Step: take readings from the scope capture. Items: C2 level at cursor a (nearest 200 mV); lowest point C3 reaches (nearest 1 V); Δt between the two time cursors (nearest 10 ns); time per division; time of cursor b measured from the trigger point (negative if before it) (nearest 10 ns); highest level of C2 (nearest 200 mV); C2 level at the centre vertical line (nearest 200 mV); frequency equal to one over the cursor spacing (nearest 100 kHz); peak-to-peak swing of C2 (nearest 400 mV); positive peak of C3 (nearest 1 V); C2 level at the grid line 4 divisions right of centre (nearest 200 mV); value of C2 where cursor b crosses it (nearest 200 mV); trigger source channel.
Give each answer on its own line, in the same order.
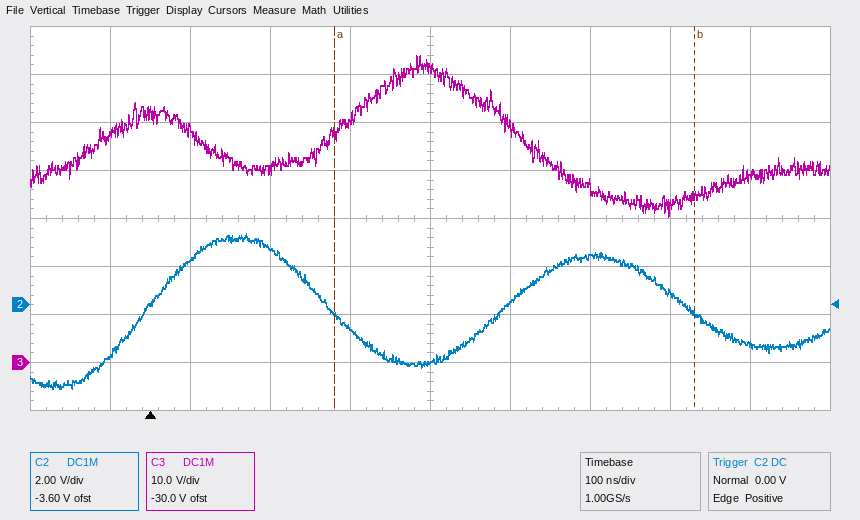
-400 mV
30 V
450 ns
100 ns
+680 ns
3.0 V
-2.4 V
2.2 MHz
6.4 V
64 V
-1.6 V
-400 mV
C2
